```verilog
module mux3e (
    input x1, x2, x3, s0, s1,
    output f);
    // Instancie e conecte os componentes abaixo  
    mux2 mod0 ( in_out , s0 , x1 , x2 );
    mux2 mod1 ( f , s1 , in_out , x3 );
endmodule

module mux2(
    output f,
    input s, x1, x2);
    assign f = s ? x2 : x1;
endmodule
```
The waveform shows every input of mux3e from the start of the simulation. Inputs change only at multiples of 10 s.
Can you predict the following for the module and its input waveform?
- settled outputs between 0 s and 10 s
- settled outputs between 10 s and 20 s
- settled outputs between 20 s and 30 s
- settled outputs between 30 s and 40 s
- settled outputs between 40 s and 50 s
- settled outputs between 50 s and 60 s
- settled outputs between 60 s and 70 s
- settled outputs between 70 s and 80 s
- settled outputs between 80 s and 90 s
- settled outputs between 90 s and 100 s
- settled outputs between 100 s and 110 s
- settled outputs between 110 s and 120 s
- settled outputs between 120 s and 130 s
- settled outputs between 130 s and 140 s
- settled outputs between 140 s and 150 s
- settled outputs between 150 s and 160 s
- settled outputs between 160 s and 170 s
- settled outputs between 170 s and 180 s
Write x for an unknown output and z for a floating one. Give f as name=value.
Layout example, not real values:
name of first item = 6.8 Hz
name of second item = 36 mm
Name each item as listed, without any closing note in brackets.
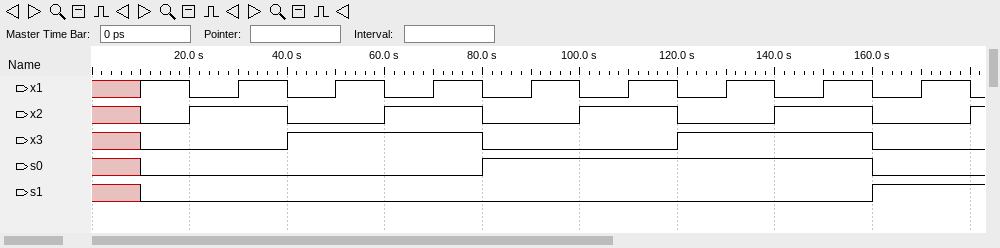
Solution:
settled outputs between 0 s and 10 s = f=x
settled outputs between 10 s and 20 s = f=1
settled outputs between 20 s and 30 s = f=0
settled outputs between 30 s and 40 s = f=1
settled outputs between 40 s and 50 s = f=0
settled outputs between 50 s and 60 s = f=1
settled outputs between 60 s and 70 s = f=0
settled outputs between 70 s and 80 s = f=1
settled outputs between 80 s and 90 s = f=0
settled outputs between 90 s and 100 s = f=0
settled outputs between 100 s and 110 s = f=1
settled outputs between 110 s and 120 s = f=1
settled outputs between 120 s and 130 s = f=0
settled outputs between 130 s and 140 s = f=0
settled outputs between 140 s and 150 s = f=1
settled outputs between 150 s and 160 s = f=1
settled outputs between 160 s and 170 s = f=0
settled outputs between 170 s and 180 s = f=0
